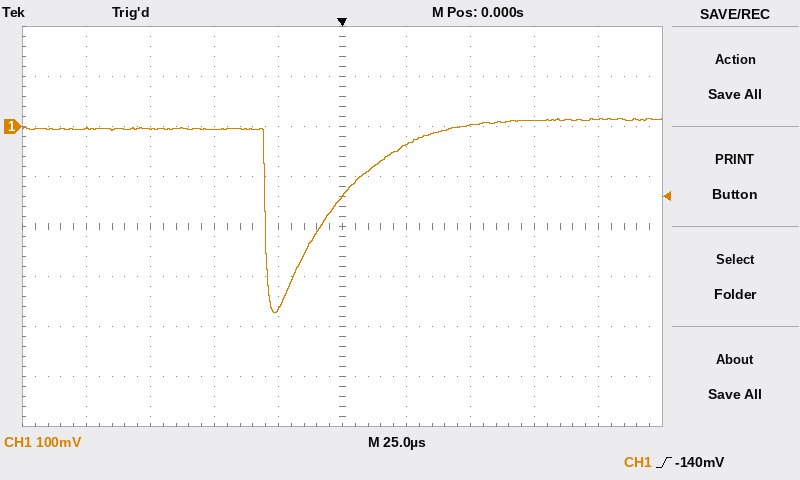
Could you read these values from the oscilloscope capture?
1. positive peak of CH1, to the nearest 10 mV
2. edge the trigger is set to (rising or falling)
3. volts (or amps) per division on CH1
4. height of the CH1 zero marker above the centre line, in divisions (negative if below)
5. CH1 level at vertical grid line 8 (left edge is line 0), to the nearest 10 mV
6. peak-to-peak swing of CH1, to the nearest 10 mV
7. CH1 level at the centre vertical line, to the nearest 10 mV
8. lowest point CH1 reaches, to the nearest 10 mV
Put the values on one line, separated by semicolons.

20 mV; rising; 100 mV; +2.0 div; 10 mV; 390 mV; -140 mV; -370 mV
